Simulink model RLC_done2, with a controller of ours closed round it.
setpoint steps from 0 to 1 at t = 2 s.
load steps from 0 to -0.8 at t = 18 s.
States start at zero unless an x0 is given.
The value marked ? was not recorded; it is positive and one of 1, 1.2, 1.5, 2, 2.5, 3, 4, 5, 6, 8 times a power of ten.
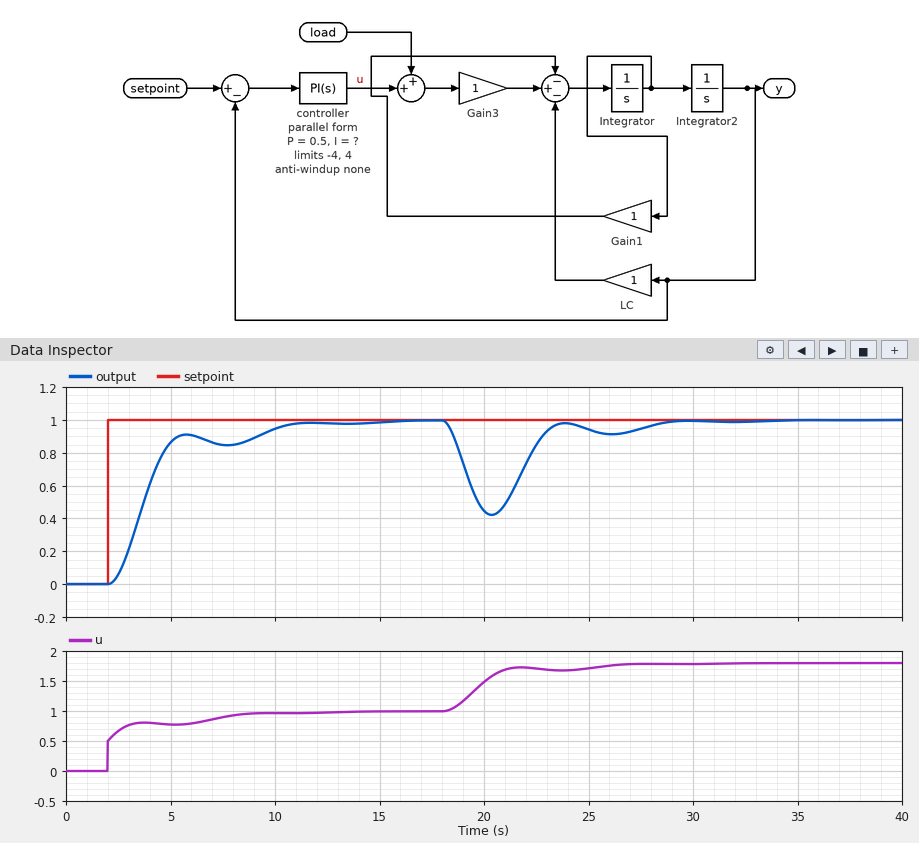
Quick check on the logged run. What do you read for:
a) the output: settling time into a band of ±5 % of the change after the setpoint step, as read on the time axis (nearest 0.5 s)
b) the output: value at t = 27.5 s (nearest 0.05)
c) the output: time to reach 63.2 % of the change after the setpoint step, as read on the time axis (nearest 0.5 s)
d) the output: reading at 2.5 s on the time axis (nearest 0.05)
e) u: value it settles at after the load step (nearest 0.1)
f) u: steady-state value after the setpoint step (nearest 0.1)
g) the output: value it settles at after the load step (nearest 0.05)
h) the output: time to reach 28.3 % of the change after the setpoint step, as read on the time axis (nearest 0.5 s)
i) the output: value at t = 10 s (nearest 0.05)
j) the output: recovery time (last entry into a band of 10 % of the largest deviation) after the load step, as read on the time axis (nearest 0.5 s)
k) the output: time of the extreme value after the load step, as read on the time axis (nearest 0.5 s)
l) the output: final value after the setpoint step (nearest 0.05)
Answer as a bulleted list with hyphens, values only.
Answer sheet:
- 10.0 s
- 0.95
- 4.0 s
- 0.05
- 1.8
- 1.0
- 1.00
- 3.0 s
- 0.95
- 27.5 s
- 20.5 s
- 1.00
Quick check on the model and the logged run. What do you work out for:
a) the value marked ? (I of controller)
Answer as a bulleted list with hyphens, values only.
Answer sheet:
- 0.4
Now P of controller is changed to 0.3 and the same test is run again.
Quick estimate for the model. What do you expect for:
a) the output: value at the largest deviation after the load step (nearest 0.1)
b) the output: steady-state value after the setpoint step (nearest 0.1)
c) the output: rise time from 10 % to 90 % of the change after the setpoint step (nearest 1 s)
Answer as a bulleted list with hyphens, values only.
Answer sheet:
- 0.4
- 1.0
- 3 s
